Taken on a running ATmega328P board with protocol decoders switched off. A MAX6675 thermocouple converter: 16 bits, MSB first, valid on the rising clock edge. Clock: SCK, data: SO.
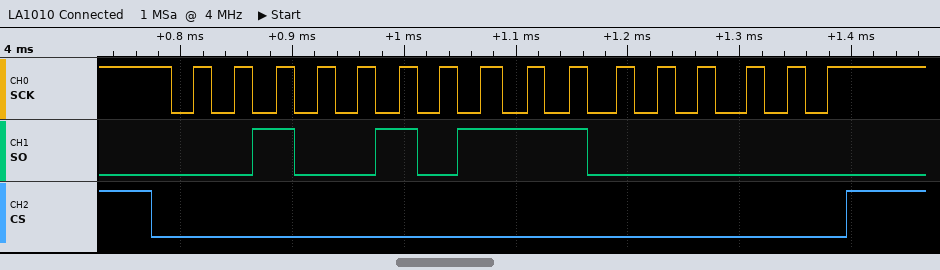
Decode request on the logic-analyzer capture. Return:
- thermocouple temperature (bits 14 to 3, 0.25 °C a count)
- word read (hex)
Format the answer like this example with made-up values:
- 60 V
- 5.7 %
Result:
- 302.00 °C
- 0x25C0
